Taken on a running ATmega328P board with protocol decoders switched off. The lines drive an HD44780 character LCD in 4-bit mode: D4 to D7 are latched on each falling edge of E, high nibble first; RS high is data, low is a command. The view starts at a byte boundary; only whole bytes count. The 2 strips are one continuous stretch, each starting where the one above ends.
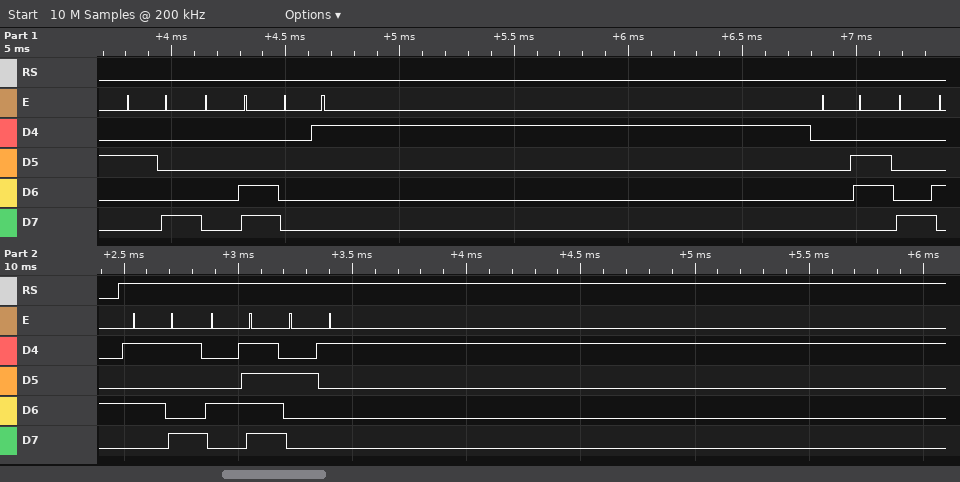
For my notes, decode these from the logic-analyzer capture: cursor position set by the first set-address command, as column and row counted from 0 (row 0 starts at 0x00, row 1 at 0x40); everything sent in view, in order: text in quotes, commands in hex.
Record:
column 4, row 0
0x28 0x0C 0x01 0x06 0x84 "YO!"
